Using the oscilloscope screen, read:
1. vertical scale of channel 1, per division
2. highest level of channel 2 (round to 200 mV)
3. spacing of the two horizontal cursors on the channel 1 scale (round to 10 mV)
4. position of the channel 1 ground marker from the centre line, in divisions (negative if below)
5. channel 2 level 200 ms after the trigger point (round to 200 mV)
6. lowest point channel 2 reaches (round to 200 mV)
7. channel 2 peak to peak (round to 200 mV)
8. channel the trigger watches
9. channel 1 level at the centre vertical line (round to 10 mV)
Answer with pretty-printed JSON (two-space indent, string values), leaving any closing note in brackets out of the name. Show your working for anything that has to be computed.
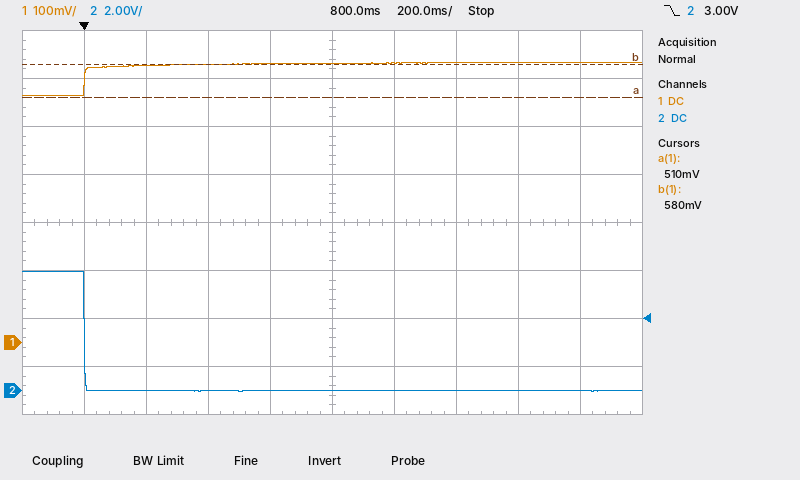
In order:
{
  "vertical scale of channel 1, per division": "100 mV",
  "highest level of channel 2": "5.0 V",
  "spacing of the two horizontal cursors on the channel 1 scale": "70 mV",
  "position of the channel 1 ground marker from the centre line, in divisions": "-2.5 div",
  "channel 2 level 200 ms after the trigger point": "0.0 V",
  "lowest point channel 2 reaches": "0.0 V",
  "channel 2 peak to peak": "5.0 V − (0.0 V) = 5.0 V",
  "channel the trigger watches": "channel 2",
  "channel 1 level at the centre vertical line": "580 mV"
}
